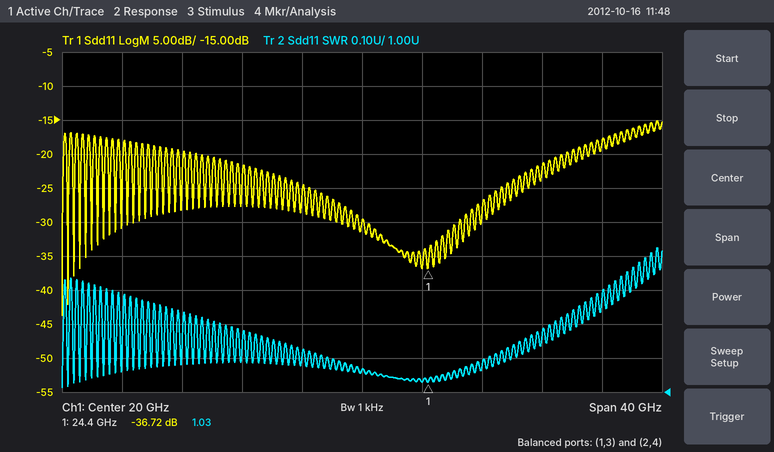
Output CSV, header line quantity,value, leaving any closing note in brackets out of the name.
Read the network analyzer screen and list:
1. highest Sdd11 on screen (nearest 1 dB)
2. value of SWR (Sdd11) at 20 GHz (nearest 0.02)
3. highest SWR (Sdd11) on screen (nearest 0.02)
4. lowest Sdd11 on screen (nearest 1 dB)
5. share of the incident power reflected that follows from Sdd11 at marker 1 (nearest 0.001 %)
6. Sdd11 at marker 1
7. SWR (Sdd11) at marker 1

quantity,value
highest Sdd11 on screen,-15 dB
value of SWR (Sdd11) at 20 GHz,1.06
highest SWR (Sdd11) on screen,1.42
lowest Sdd11 on screen,-44 dB
share of the incident power reflected that follows from Sdd11 at marker 1,0.021 %
Sdd11 at marker 1,-36.72 dB
SWR (Sdd11) at marker 1,1.03
